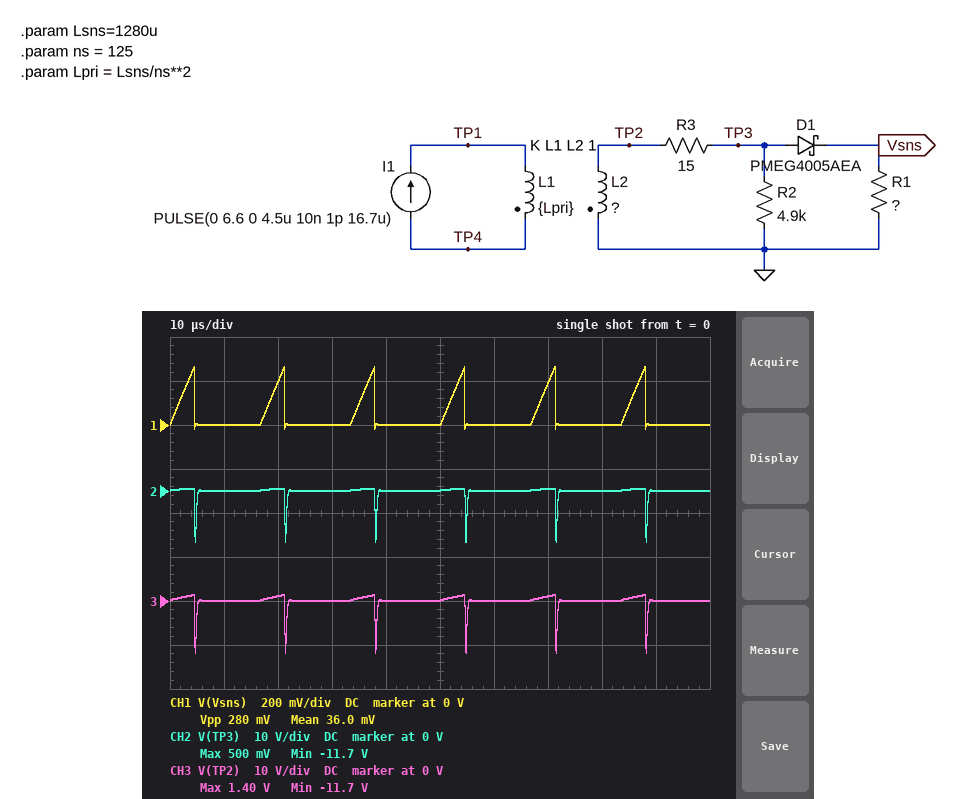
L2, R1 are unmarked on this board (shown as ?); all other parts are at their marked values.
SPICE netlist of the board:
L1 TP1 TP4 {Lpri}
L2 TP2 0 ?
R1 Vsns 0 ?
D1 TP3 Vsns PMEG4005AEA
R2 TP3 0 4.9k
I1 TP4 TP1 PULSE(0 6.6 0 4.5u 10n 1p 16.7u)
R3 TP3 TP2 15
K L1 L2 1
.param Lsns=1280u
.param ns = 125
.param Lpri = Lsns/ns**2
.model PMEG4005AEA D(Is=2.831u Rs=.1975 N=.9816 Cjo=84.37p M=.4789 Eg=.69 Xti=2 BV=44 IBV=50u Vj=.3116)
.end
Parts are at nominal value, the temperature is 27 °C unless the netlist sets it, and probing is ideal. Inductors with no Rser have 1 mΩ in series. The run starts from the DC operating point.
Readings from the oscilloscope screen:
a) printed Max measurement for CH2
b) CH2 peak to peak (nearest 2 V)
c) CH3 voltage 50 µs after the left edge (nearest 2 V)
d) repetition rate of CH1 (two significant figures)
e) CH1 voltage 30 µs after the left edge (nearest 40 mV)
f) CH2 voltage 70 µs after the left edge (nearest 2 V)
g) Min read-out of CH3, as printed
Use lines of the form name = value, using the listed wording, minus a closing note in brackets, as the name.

printed Max measurement for CH2 = 500 mV
CH2 peak to peak = 12 V
CH3 voltage 50 µs after the left edge = 0 V
repetition rate of CH1 = 60 kHz
CH1 voltage 30 µs after the left edge = 0 V
CH2 voltage 70 µs after the left edge = 0 V
Min read-out of CH3, as printed = -11.7 V
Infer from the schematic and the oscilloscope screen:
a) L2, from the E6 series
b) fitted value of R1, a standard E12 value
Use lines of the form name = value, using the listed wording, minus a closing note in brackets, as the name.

L2, from the E6 series = 1 mH
fitted value of R1, a standard E12 value = 4.7 Ω
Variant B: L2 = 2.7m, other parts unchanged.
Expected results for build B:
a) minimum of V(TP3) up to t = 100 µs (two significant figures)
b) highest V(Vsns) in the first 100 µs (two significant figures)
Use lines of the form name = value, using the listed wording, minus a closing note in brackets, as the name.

minimum of V(TP3) up to t = 100 µs = -3.4 V
highest V(Vsns) in the first 100 µs = 170 mV
